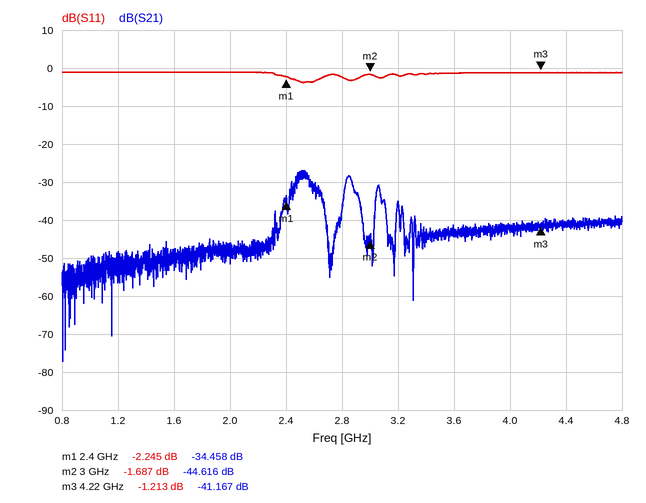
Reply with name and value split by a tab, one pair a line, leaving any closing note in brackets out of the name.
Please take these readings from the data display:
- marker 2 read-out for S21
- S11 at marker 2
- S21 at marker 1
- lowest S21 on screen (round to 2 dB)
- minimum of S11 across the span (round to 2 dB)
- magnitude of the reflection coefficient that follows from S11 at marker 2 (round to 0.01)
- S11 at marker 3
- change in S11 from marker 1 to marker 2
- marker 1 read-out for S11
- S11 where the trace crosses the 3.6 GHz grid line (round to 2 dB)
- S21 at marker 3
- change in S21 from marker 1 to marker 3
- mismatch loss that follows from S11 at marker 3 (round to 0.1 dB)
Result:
marker 2 read-out for S21	-44.616 dB
S11 at marker 2	-1.687 dB
S21 at marker 1	-34.458 dB
lowest S21 on screen	-78 dB
minimum of S11 across the span	-4 dB
magnitude of the reflection coefficient that follows from S11 at marker 2	0.82
S11 at marker 3	-1.213 dB
change in S11 from marker 1 to marker 2	0.558 dB
marker 1 read-out for S11	-2.245 dB
S11 where the trace crosses the 3.6 GHz grid line	-2 dB
S21 at marker 3	-41.167 dB
change in S21 from marker 1 to marker 3	-6.709 dB
mismatch loss that follows from S11 at marker 3	6.1 dB
